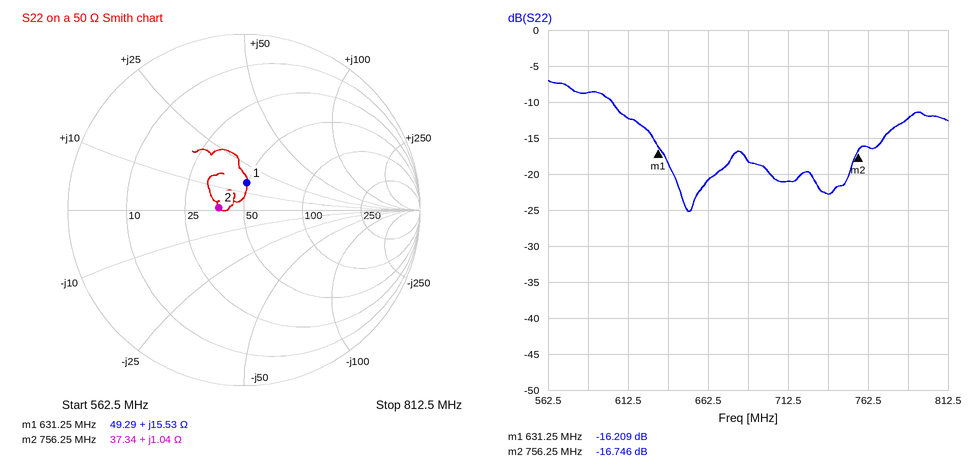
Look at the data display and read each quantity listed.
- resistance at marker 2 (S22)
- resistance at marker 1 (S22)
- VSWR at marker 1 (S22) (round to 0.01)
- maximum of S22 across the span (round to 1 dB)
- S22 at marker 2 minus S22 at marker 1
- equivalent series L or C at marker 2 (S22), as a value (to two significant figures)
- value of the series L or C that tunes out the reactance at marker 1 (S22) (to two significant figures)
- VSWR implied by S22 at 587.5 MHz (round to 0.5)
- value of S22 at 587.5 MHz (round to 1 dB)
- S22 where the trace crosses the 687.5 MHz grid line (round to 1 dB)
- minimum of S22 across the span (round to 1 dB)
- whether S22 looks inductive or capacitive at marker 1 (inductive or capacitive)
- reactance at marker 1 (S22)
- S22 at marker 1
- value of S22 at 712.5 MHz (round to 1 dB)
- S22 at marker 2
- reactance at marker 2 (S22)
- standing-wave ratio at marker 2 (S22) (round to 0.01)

37.34 Ω
49.29 Ω
1.37
-7 dB
-0.537 dB
220 pH
16 pF
2.0
-9 dB
-18 dB
-25 dB
inductive
+15.53 Ω
-16.209 dB
-21 dB
-16.746 dB
+1.04 Ω
1.34
